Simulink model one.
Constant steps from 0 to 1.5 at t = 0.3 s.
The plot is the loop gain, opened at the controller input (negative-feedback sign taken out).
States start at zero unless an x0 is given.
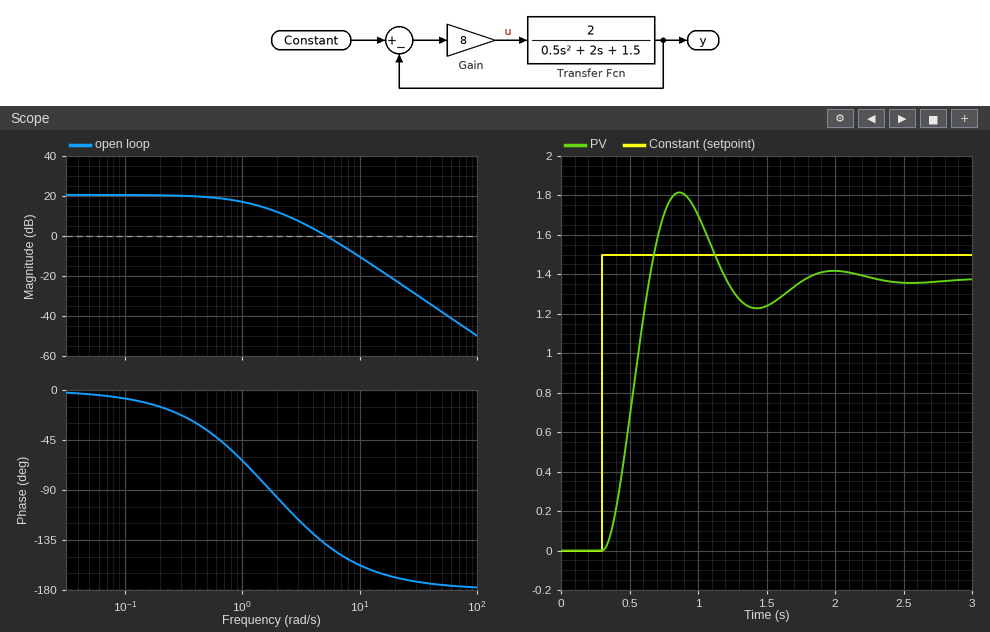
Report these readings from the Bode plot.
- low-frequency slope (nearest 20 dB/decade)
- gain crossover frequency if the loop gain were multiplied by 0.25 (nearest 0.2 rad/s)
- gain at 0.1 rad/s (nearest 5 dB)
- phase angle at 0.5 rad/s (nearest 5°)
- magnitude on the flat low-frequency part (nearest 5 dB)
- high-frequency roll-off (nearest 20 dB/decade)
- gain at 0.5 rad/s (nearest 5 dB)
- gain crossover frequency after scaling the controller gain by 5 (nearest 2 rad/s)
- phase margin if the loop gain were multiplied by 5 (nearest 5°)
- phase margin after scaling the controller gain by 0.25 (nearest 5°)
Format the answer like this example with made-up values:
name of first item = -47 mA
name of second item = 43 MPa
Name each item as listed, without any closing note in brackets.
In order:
low-frequency slope = 0 dB/decade
gain crossover frequency if the loop gain were multiplied by 0.25 = 2.0 rad/s
gain at 0.1 rad/s = 20 dB
phase angle at 0.5 rad/s = -35°
magnitude on the flat low-frequency part = 20 dB
high-frequency roll-off = -40 dB/decade
gain at 0.5 rad/s = 20 dB
gain crossover frequency after scaling the controller gain by 5 = 12 rad/s
phase margin if the loop gain were multiplied by 5 = 20°
phase margin after scaling the controller gain by 0.25 = 85°
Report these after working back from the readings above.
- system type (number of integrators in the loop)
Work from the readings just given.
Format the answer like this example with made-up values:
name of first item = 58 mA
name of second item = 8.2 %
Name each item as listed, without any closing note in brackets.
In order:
system type = 0
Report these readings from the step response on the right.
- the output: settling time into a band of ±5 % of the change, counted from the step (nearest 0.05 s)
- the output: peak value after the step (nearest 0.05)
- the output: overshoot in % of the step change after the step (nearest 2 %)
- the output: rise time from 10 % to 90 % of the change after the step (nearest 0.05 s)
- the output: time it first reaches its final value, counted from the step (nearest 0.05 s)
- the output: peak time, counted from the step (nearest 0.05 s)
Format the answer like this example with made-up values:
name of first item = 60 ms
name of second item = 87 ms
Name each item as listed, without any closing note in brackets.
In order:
the output: settling time into a band of ±5 % of the change, counted from the step = 1.35 s
the output: peak value after the step = 1.80
the output: overshoot in % of the step change after the step = 32 %
the output: rise time from 10 % to 90 % of the change after the step = 0.25 s
the output: time it first reaches its final value, counted from the step = 0.35 s
the output: peak time, counted from the step = 0.55 s
